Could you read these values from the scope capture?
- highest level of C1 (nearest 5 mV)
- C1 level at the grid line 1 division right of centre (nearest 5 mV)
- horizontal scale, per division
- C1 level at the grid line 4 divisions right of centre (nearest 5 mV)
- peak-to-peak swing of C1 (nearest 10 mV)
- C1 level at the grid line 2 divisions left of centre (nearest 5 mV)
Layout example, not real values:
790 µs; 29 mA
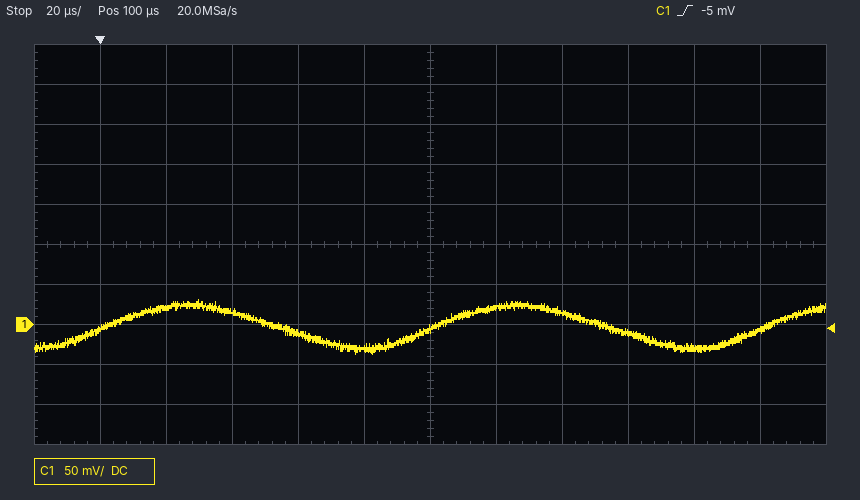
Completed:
30 mV; 20 mV; 20 µs; -30 mV; 70 mV; -10 mV
